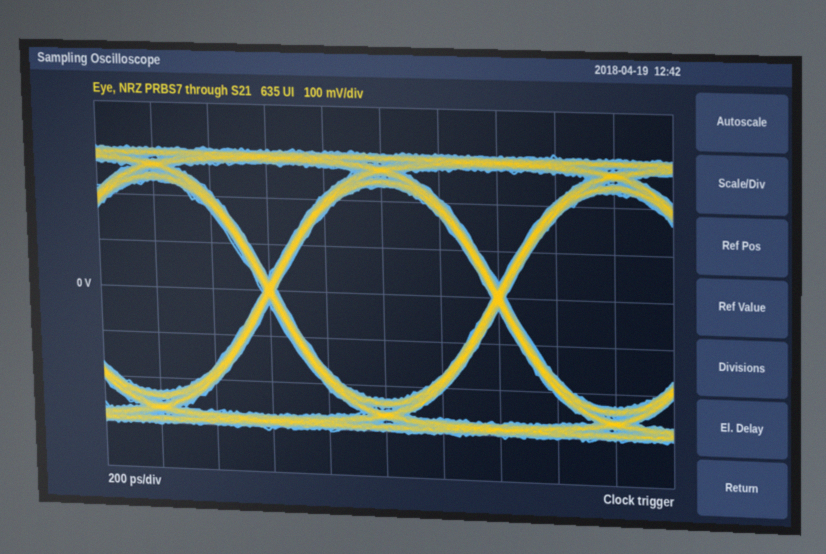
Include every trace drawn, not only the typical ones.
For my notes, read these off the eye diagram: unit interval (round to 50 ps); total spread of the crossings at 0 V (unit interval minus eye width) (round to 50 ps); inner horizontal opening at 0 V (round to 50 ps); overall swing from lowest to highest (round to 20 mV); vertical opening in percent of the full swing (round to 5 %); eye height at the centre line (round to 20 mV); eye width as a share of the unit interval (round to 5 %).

800 ps
50 ps
750 ps
620 mV
75 %
460 mV
95 %
